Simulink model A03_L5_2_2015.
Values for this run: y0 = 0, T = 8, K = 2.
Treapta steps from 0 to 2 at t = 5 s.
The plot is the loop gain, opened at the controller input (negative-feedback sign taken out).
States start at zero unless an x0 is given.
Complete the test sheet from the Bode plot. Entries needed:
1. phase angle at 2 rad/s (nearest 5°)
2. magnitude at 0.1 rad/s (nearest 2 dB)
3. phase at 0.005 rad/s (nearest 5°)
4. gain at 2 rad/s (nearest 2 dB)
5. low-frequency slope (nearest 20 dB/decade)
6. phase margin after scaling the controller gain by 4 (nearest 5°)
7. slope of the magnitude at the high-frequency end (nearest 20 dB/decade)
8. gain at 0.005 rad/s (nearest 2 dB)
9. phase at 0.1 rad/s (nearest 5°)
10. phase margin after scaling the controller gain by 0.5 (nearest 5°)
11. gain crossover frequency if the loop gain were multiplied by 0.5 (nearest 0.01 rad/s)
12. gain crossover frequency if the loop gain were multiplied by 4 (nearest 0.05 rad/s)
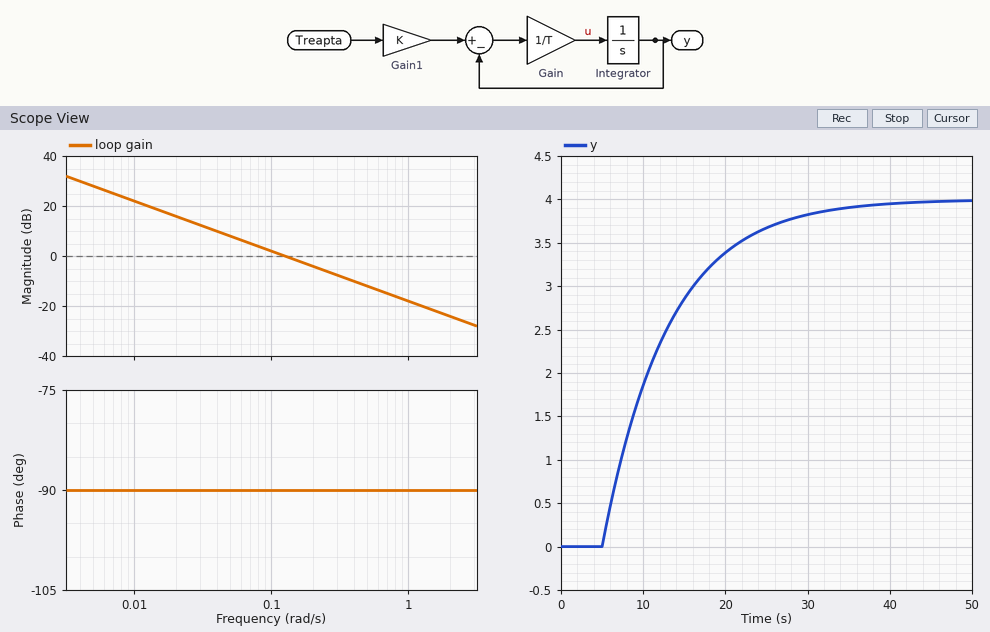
-90°
2 dB
-90°
-24 dB
-20 dB/decade
90°
-20 dB/decade
28 dB
-90°
90°
0.06 rad/s
0.50 rad/s
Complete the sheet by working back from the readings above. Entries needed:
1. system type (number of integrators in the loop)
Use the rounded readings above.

1
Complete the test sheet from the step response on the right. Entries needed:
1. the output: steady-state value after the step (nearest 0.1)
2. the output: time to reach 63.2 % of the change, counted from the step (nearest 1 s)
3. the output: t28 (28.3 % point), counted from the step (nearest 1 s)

4.0
8 s
3 s
